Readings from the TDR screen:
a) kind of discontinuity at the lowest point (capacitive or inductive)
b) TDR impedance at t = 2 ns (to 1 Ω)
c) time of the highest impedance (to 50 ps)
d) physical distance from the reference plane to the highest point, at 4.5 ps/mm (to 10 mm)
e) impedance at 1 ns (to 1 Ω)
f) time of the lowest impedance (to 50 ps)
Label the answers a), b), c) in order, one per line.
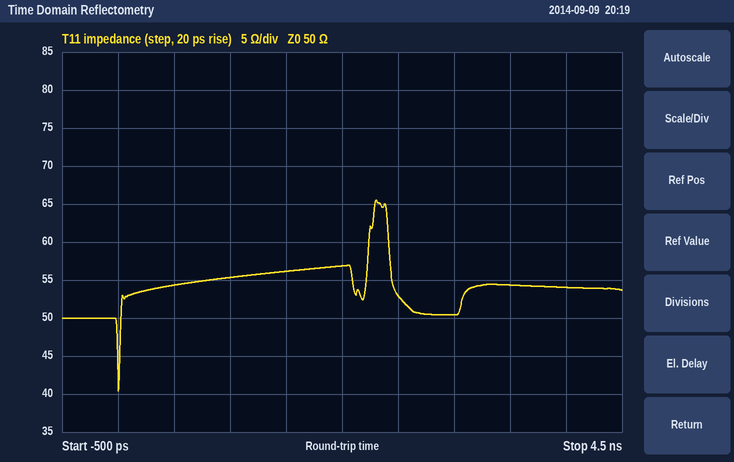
a) capacitive
b) 57 Ω
c) 2.30 ns
d) 260 mm
e) 55 Ω
f) 0 ps
